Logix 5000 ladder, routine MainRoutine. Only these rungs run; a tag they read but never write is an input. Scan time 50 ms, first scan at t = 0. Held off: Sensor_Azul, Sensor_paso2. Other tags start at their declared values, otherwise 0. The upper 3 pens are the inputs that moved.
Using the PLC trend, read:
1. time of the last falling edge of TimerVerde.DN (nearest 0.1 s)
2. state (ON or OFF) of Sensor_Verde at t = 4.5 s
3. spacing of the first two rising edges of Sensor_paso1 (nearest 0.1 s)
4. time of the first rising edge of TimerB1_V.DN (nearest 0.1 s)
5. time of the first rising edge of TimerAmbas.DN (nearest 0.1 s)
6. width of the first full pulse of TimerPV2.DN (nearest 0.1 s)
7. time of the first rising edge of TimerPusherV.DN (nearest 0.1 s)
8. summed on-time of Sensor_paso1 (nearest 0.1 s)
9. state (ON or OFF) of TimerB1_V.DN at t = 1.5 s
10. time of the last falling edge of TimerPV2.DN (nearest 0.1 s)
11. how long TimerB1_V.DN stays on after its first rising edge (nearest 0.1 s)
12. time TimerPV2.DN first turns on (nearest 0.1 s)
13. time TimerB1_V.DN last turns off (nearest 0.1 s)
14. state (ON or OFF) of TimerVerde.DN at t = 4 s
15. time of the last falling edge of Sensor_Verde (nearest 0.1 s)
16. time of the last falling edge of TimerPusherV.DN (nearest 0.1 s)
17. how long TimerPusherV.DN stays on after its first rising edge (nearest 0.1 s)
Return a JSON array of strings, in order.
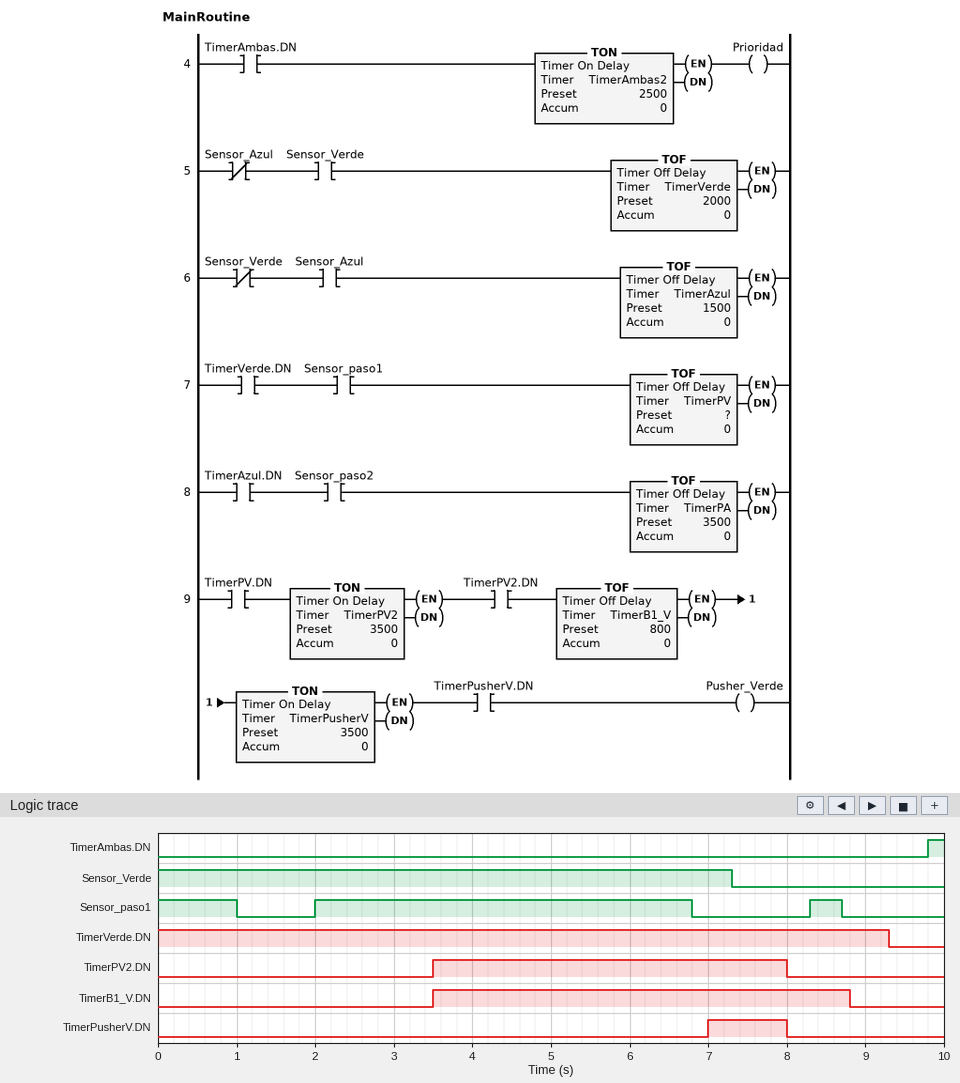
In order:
["9.3 s", "ON", "6.3 s", "3.5 s", "9.8 s", "4.5 s", "7.0 s", "6.2 s", "OFF", "8.0 s", "5.3 s", "3.5 s", "8.8 s", "ON", "7.3 s", "8.0 s", "1.0 s"]
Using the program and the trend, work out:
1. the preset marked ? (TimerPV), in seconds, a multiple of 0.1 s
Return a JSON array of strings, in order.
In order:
["1.2 s"]
